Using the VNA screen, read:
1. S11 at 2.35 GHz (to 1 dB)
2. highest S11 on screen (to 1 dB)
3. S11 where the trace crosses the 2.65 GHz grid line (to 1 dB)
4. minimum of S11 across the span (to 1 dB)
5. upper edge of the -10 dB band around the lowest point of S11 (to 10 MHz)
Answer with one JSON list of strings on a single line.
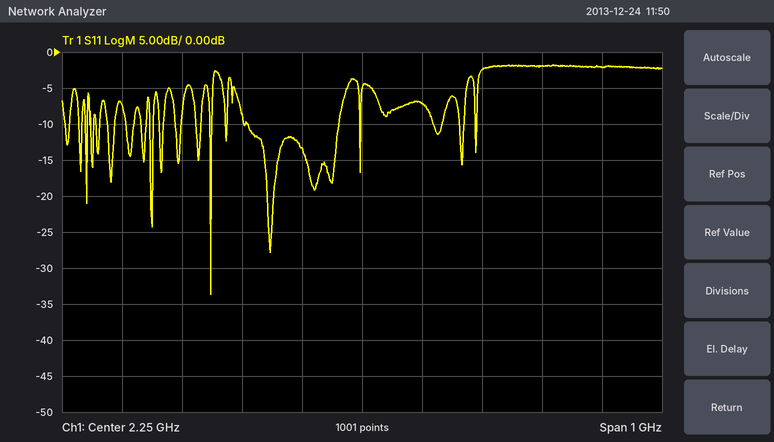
["-7 dB", "-2 dB", "-2 dB", "-34 dB", "2.00 GHz"]
